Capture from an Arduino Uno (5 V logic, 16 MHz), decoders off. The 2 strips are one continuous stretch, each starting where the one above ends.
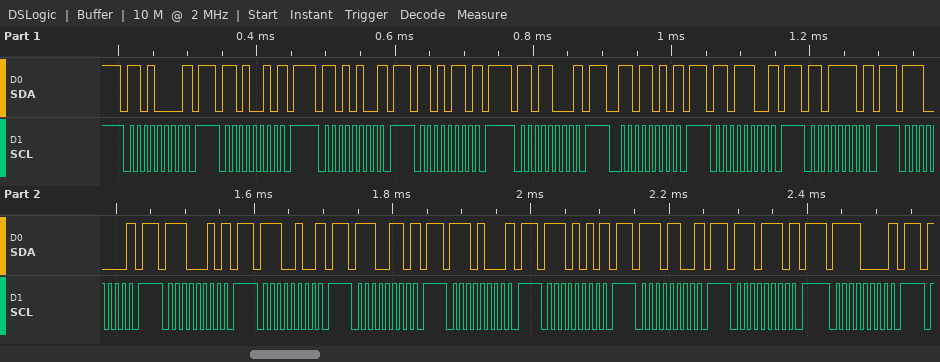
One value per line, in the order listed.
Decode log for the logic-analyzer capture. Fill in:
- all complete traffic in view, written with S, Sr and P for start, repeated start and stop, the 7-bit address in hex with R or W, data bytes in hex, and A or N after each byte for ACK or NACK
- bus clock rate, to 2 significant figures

S 68W N P S 69W N P S 6AW N P S 6BW N P S 6CW N P S 6DW N P S 6EW N P S 6FW N P S 70W N P S 71W N P S 72W N P S 73W N P S 74W N P S 75W N P S 76W N P S 77W N P S 78W N P
100 kHz
